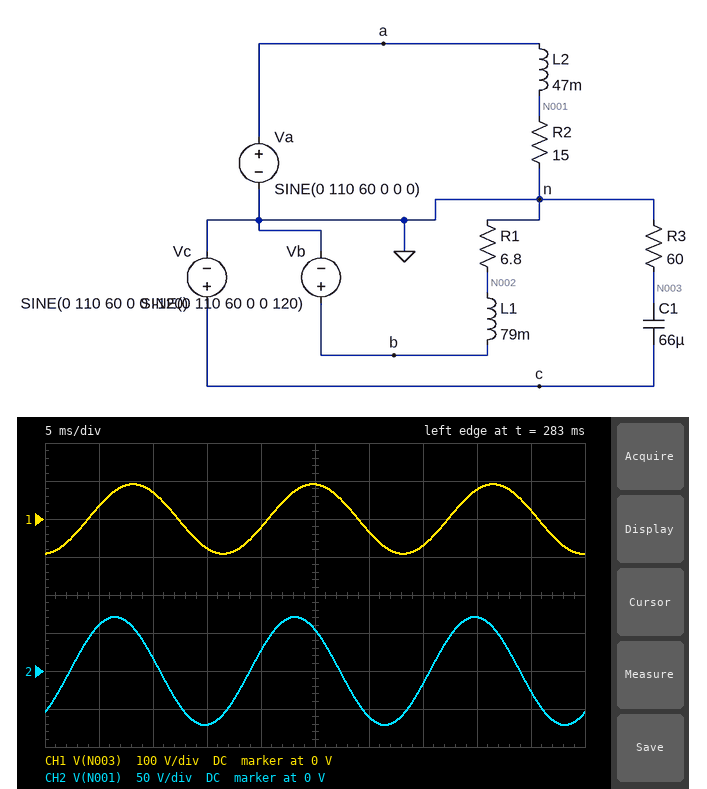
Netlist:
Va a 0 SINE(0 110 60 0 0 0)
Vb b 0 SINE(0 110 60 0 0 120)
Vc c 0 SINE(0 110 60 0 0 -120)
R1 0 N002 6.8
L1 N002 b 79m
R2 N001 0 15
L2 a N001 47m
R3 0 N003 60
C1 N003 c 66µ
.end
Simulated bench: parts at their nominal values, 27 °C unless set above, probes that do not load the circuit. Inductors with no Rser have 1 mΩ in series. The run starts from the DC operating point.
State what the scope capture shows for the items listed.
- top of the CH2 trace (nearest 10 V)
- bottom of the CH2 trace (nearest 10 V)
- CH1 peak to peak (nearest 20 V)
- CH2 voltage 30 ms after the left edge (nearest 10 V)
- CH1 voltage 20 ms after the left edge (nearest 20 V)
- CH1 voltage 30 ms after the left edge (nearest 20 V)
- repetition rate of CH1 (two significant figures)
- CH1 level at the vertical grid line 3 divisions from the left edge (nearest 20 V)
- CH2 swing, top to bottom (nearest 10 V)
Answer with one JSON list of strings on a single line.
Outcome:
["70 V", "-70 V", "180 V", "-60 V", "-20 V", "-40 V", "60 Hz", "-80 V", "140 V"]
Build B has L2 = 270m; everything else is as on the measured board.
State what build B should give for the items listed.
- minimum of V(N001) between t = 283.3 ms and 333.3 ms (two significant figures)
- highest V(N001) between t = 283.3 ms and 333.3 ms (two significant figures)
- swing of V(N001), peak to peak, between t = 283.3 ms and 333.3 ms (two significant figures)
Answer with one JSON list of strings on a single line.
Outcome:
["-16 V", "16 V", "32 V"]
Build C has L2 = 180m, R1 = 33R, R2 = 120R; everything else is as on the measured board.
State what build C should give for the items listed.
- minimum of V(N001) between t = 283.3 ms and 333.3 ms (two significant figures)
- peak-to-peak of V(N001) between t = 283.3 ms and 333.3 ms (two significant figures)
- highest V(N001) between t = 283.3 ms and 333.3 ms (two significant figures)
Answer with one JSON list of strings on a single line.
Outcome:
["-96 V", "190 V", "96 V"]
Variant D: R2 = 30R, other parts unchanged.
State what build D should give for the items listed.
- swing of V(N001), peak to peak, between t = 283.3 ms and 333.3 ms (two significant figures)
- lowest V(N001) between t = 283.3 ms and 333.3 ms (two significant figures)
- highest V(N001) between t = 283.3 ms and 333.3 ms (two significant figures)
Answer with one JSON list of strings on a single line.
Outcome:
["190 V", "-95 V", "95 V"]
